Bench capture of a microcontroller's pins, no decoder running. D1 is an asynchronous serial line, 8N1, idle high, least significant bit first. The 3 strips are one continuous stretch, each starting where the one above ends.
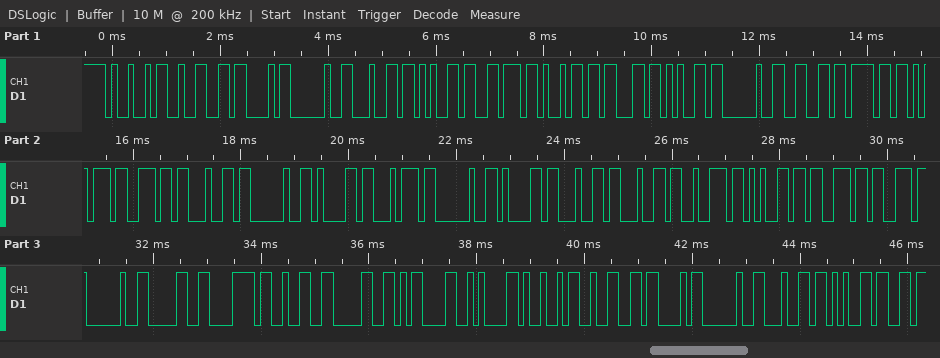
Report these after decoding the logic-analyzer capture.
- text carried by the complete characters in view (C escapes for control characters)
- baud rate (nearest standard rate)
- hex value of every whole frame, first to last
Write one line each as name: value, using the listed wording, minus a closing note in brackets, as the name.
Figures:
text carried by the complete characters in view: "I2C device found at address 0x20\r\nI2C de"
baud rate: 9600 baud
hex value of every whole frame, first to last: 49 32 43 20 64 65 76 69 63 65 20 66 6F 75 6E 64 20 61 74 20 61 64 64 72 65 73 73 20 30 78 32 30 0D 0A 49 32 43 20 64 65
